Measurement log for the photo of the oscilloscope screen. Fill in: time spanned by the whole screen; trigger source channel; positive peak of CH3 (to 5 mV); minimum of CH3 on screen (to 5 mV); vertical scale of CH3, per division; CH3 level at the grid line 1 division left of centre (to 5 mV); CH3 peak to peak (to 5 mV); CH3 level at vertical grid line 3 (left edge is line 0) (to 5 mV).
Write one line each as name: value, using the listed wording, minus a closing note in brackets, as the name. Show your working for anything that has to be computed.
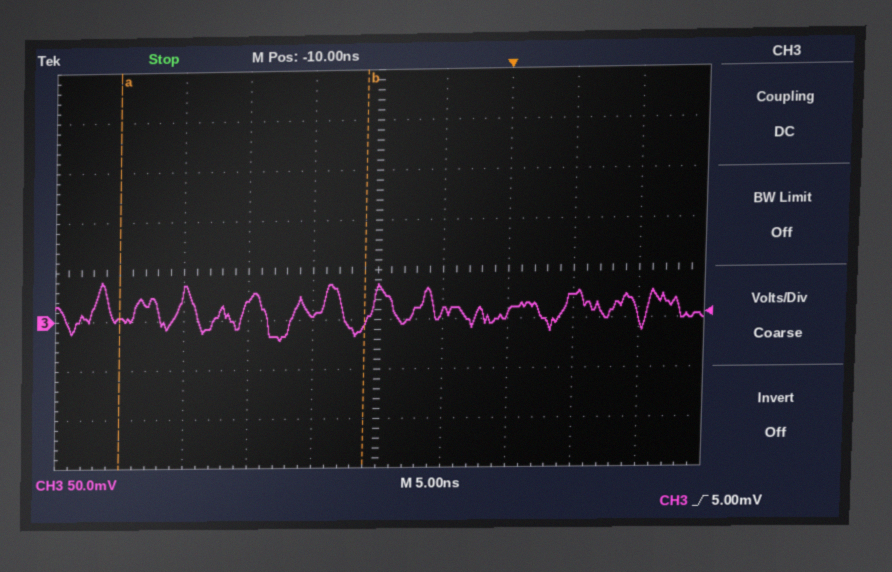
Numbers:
time spanned by the whole screen: 50 ns
trigger source channel: CH3
positive peak of CH3: 40 mV
minimum of CH3 on screen: -20 mV
vertical scale of CH3, per division: 50 mV
CH3 level at the grid line 1 division left of centre: 5 mV
CH3 peak to peak: 40 mV − (-20 mV) = 60 mV
CH3 level at vertical grid line 3 (left edge is line 0): 20 mV
